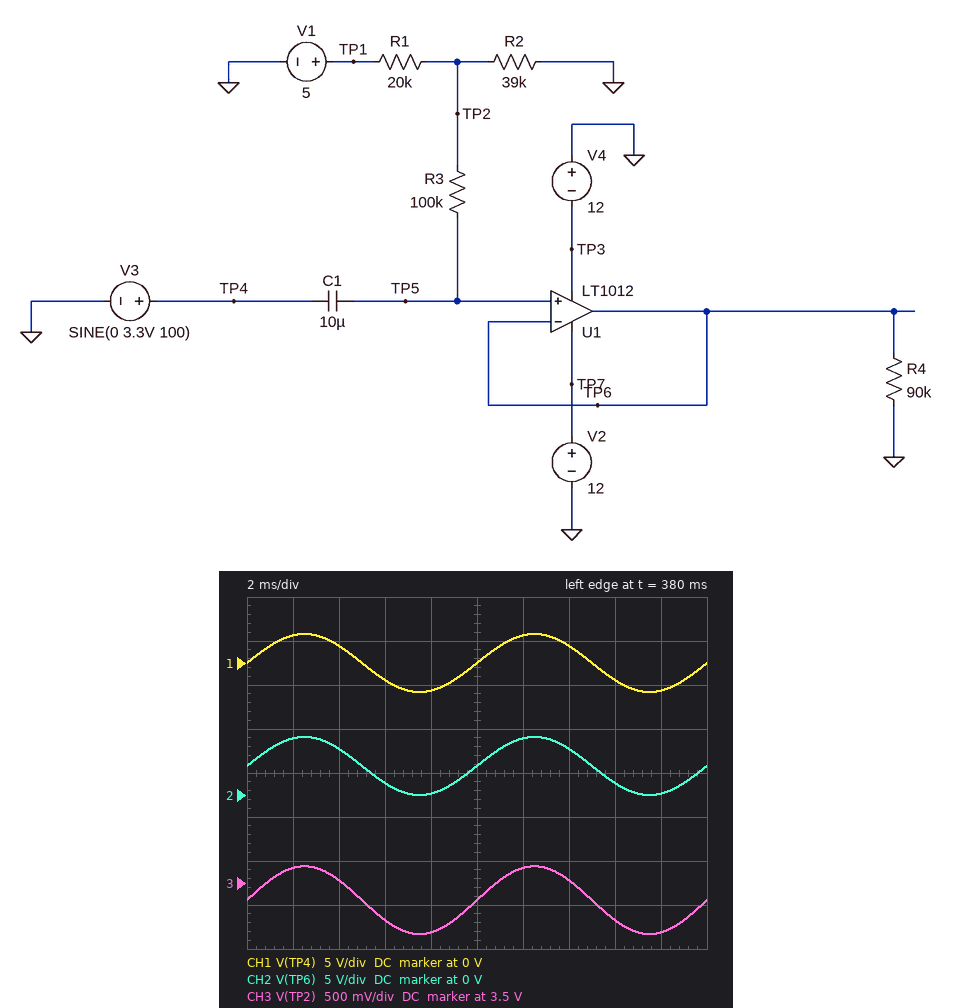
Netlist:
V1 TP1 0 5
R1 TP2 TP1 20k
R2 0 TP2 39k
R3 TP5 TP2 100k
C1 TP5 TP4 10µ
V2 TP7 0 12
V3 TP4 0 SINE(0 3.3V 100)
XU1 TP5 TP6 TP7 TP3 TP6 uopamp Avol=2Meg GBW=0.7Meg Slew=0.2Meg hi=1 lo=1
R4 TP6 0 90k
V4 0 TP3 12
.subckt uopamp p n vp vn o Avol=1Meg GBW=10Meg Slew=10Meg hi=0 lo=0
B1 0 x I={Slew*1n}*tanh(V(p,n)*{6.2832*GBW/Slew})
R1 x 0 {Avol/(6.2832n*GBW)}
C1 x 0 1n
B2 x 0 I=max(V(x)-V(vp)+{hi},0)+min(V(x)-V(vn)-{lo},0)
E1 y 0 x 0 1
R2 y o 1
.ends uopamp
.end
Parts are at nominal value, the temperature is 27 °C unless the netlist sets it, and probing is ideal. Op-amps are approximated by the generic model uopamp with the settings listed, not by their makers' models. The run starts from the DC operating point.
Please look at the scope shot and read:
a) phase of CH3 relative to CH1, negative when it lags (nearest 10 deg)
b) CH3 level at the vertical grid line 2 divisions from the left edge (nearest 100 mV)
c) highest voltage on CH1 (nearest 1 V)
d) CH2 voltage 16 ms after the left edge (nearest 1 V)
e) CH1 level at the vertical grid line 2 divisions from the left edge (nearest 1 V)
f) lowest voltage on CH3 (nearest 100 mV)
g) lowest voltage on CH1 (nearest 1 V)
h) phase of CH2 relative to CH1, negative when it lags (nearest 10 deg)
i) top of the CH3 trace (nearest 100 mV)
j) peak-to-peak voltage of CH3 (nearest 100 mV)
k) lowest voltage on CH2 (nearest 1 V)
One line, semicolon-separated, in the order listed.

0 deg; 3.5 V; 3 V; 1 V; 2 V; 2.9 V; -3 V; 0 deg; 3.7 V; 800 mV; 0 V
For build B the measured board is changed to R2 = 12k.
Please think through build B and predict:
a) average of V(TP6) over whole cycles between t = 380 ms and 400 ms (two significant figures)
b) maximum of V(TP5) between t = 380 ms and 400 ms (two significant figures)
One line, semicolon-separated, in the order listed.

1.9 V; 5.2 V
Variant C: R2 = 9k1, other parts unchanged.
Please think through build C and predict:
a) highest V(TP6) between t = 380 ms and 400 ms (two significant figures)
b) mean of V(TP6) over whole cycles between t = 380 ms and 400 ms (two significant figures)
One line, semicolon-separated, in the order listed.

4.9 V; 1.6 V
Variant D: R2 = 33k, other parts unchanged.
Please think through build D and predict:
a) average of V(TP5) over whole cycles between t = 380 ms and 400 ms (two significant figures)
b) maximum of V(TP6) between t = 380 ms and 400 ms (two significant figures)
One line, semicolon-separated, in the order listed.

3.1 V; 6.4 V
